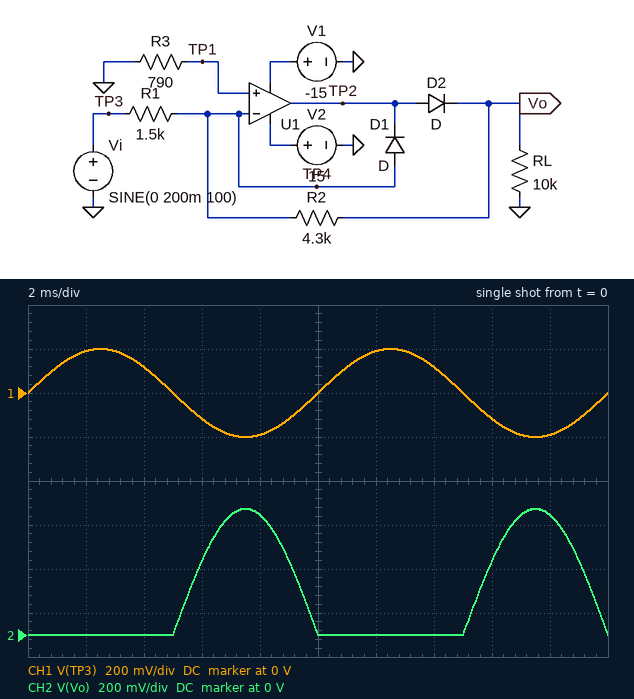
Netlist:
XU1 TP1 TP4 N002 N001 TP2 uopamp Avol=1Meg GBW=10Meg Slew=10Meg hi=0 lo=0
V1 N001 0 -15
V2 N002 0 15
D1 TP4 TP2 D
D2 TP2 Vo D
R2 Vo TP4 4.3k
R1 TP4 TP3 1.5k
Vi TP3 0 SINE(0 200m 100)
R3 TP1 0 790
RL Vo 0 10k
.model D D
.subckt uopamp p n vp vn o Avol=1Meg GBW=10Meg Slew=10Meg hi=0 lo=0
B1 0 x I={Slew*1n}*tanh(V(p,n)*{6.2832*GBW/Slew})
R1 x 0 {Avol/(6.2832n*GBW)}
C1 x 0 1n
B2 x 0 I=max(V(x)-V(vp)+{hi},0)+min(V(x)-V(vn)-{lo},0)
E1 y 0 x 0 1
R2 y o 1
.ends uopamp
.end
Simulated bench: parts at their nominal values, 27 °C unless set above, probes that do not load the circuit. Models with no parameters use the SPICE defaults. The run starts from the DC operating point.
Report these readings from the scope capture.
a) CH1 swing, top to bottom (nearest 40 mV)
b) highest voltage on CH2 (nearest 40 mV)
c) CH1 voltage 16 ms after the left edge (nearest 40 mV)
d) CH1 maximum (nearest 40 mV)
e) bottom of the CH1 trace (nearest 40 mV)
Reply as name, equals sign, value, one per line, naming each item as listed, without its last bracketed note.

CH1 swing, top to bottom = 400 mV
highest voltage on CH2 = 560 mV
CH1 voltage 16 ms after the left edge = -120 mV
CH1 maximum = 200 mV
bottom of the CH1 trace = -200 mV
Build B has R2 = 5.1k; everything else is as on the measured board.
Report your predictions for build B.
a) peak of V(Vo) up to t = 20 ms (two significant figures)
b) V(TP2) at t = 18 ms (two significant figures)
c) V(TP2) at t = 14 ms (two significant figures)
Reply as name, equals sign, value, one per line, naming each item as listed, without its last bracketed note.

peak of V(Vo) up to t = 20 ms = 680 mV
V(TP2) at t = 18 ms = 1.3 V
V(TP2) at t = 14 ms = -590 mV
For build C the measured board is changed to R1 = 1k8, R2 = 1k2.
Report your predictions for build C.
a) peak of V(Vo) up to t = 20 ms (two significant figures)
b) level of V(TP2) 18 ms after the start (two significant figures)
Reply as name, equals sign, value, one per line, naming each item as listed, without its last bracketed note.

peak of V(Vo) up to t = 20 ms = 130 mV
level of V(TP2) 18 ms after the start = 730 mV
